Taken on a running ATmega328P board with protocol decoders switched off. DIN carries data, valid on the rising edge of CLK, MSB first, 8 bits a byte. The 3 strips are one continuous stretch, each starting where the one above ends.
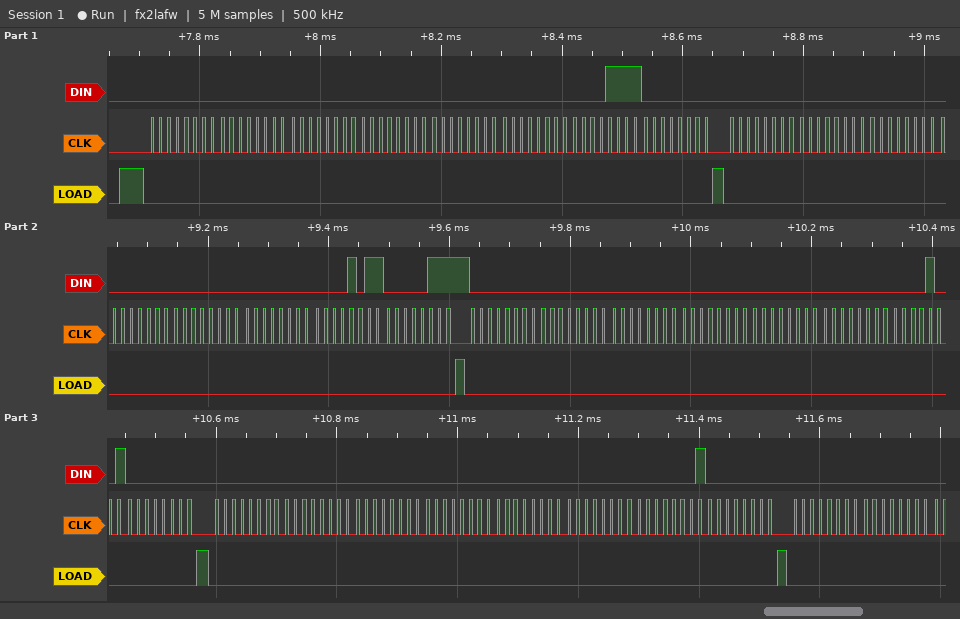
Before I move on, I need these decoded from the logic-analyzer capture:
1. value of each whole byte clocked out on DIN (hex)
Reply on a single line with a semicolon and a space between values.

00 00 00 00 00 00 0F 00 00 00 00 00 00 00 0B 07 00 00 00 00 00 00 09 00 00 00 00 00 00 00 01 00 00 00
